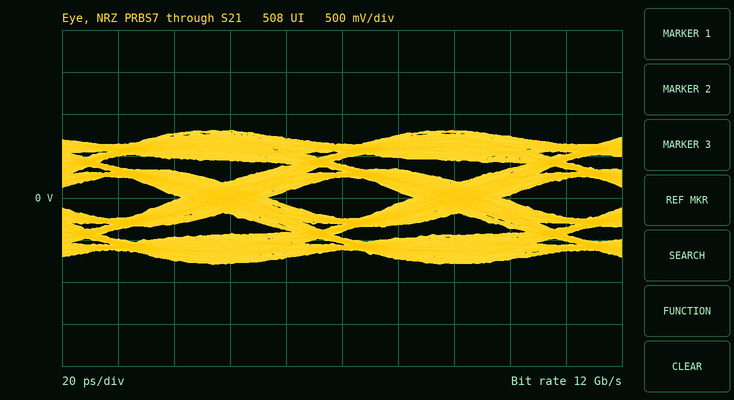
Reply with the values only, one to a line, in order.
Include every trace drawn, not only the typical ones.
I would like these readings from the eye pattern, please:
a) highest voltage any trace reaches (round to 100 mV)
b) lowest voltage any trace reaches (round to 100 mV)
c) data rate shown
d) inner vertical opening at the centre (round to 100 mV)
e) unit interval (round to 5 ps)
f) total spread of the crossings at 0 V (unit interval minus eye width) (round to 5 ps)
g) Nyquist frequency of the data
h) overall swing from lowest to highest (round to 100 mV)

800 mV
-800 mV
12 Gb/s
500 mV
85 ps
30 ps
6 GHz
1.6 V
